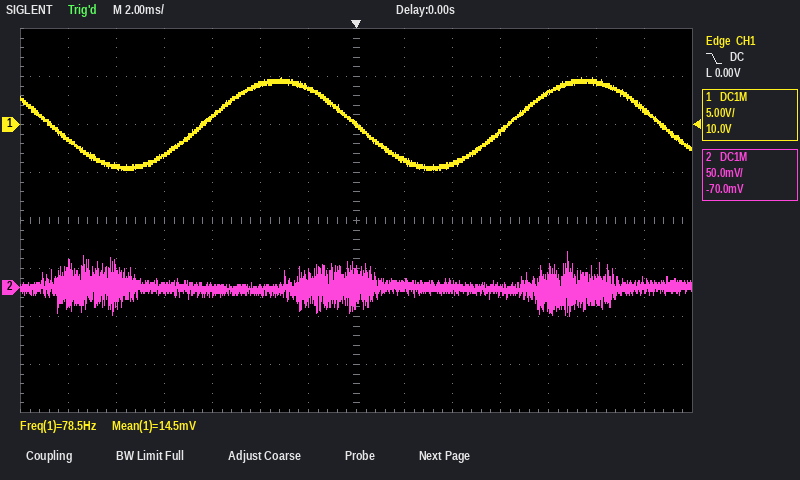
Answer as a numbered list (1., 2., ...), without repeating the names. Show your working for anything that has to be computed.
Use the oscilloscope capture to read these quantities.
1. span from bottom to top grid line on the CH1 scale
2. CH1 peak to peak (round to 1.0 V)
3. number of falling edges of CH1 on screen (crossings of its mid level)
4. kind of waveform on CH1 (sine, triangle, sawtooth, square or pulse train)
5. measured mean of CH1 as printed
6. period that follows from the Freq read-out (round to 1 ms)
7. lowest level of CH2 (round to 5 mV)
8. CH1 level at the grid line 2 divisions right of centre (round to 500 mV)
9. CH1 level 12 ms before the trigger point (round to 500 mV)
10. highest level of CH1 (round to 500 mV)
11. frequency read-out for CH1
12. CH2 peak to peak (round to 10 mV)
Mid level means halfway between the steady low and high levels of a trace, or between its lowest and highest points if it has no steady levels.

1. 40 V
2. 10.0 V
3. 3
4. sine
5. 14.5 mV
6. 1 / 78.5 Hz ≈ 13 ms
7. -30 mV
8. -4.0 V
9. -1.5 V
10. 5.0 V
11. 78.5 Hz
12. 70 mV
